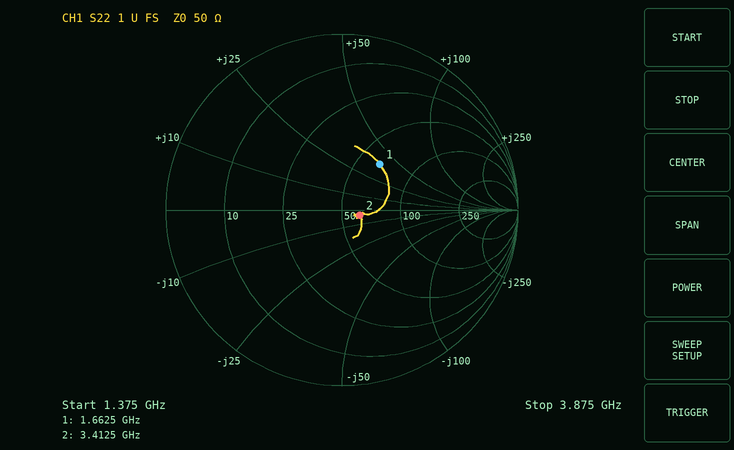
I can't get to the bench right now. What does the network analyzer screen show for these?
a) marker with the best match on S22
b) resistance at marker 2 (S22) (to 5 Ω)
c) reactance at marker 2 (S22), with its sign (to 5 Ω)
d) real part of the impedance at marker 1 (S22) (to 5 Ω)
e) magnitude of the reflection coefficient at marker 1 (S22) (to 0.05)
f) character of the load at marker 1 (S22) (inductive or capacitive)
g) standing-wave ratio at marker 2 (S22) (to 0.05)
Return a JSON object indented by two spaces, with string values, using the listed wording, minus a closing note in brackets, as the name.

{
  "marker with the best match on S22": "marker 2",
  "resistance at marker 2 (S22)": "60 Ω",
  "reactance at marker 2 (S22), with its sign": "-5 Ω",
  "real part of the impedance at marker 1 (S22)": "65 Ω",
  "magnitude of the reflection coefficient at marker 1 (S22)": "0.35",
  "character of the load at marker 1 (S22)": "inductive",
  "standing-wave ratio at marker 2 (S22)": "1.25"
}
